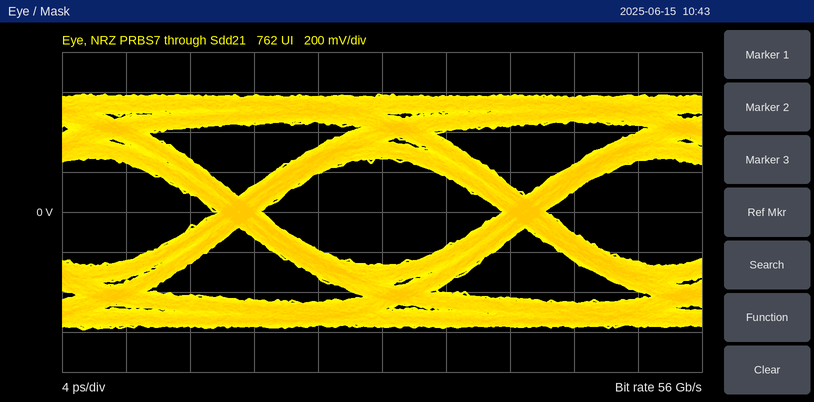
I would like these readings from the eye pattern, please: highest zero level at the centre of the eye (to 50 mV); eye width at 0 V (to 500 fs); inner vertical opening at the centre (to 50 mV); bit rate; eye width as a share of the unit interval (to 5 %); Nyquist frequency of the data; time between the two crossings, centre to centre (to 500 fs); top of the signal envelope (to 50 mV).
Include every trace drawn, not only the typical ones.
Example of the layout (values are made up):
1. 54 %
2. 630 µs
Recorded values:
1. -250 mV
2. 15.0 ps
3. 550 mV
4. 56 Gb/s
5. 85 %
6. 28 GHz
7. 18.0 ps
8. 600 mV
